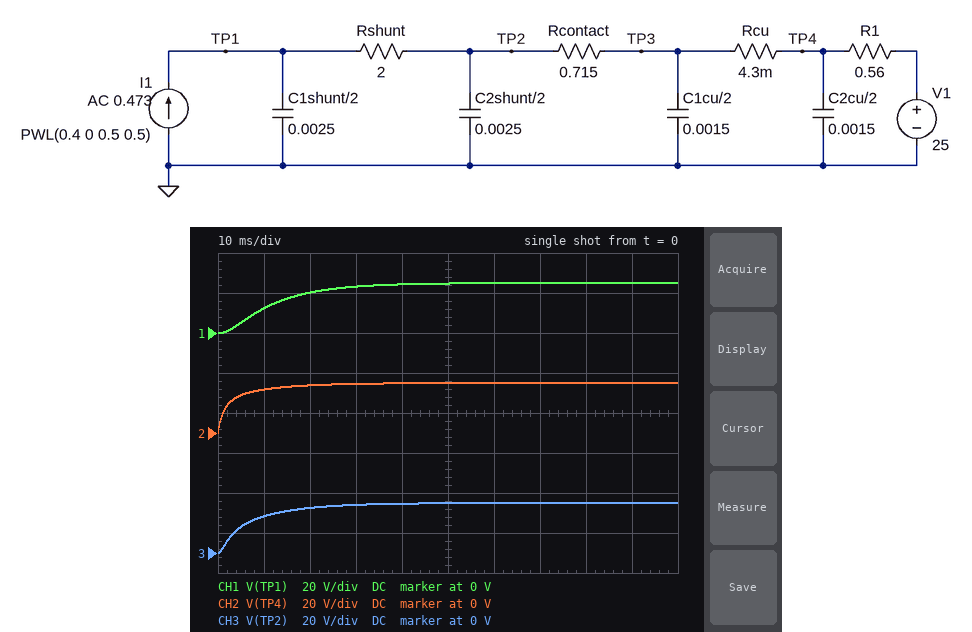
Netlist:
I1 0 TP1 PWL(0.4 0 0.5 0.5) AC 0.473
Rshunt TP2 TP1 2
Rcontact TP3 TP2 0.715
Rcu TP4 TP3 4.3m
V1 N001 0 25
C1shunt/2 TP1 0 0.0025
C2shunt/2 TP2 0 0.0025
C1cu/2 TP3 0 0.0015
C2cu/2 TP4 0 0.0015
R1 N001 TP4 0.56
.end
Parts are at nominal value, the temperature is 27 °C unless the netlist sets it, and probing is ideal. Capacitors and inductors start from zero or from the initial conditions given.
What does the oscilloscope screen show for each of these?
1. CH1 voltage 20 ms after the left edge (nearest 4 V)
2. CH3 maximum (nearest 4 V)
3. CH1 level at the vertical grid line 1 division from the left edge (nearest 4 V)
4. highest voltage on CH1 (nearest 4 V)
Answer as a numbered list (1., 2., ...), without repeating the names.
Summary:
1. 20 V
2. 24 V
3. 12 V
4. 24 V
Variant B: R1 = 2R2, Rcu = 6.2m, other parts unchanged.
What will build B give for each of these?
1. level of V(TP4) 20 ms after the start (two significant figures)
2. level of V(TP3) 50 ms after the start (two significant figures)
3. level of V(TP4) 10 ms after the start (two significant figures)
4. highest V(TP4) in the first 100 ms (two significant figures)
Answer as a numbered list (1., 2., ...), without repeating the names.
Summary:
1. 17 V
2. 23 V
3. 13 V
4. 25 V
